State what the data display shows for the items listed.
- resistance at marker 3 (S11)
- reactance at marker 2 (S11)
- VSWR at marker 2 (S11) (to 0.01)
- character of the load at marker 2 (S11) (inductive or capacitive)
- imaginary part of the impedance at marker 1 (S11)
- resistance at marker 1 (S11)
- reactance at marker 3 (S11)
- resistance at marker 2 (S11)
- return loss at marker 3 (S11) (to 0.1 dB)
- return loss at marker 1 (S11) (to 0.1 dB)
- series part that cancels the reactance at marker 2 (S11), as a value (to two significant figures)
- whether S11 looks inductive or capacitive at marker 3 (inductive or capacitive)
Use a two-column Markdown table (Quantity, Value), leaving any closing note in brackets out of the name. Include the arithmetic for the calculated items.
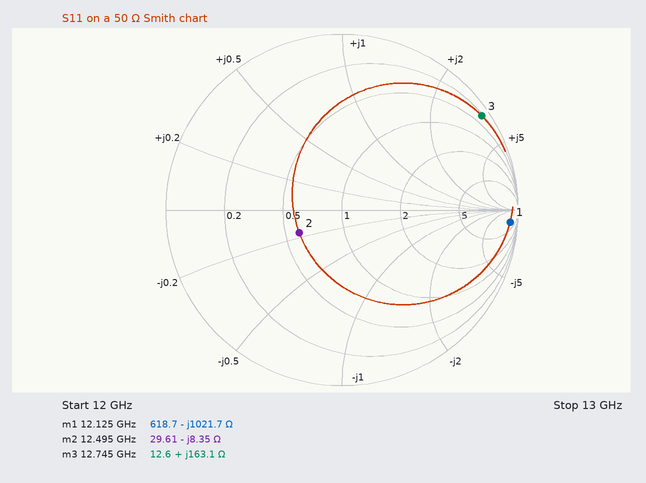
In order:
| Quantity | Value |
|---|---|
| resistance at marker 3 | 12.6 Ω |
| reactance at marker 2 | -8.35 Ω |
| VSWR at marker 2 (S11) | 1.76 |
| character of the load at marker 2 (S11) | capacitive |
| imaginary part of the impedance at marker 1 | -1021.7 Ω |
| resistance at marker 1 | 618.7 Ω |
| reactance at marker 3 | +163.1 Ω |
| resistance at marker 2 | 29.61 Ω |
| return loss at marker 3 (S11) | 0.4 dB |
| return loss at marker 1 (S11) | 0.4 dB |
| series part that cancels the reactance at marker 2 (S11), as a value | L = 8.35 Ω/(2π × 12.495 GHz) ≈ 106 pH, so 110 pH to two significant figures |
| whether S11 looks inductive or capacitive at marker 3 | inductive |
